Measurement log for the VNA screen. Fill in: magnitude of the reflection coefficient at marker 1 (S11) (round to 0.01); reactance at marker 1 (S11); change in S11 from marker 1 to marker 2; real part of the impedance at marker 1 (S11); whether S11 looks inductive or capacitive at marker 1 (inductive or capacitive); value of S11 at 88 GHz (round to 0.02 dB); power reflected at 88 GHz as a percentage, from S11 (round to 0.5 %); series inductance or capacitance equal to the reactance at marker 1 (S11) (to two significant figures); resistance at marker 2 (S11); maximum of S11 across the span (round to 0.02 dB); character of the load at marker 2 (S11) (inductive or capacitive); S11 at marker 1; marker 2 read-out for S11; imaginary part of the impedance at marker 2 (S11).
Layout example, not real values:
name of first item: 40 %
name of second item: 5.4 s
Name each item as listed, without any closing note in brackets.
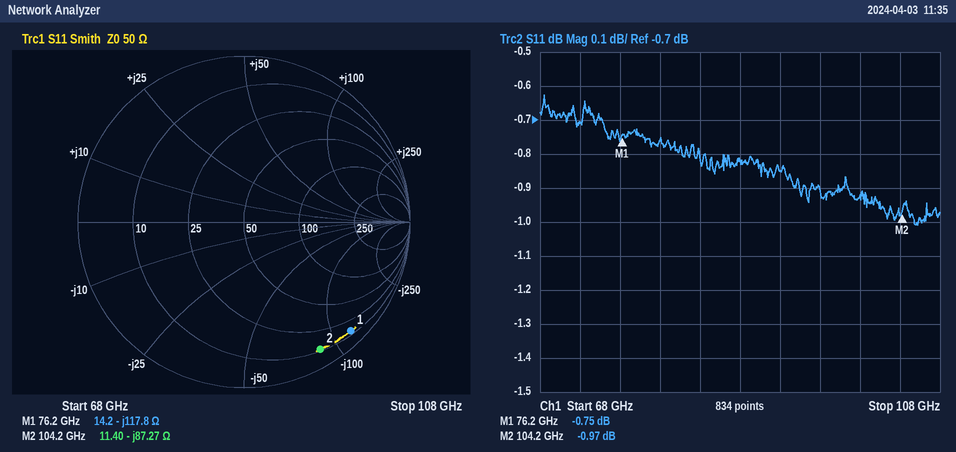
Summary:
magnitude of the reflection coefficient at marker 1 (S11): 0.92
reactance at marker 1: -117.8 Ω
change in S11 from marker 1 to marker 2: -0.22 dB
real part of the impedance at marker 1: 14.2 Ω
whether S11 looks inductive or capacitive at marker 1: capacitive
value of S11 at 88 GHz: -0.82 dB
power reflected at 88 GHz as a percentage, from S11: 83.0 %
series inductance or capacitance equal to the reactance at marker 1 (S11): 18 fF
resistance at marker 2: 11.40 Ω
maximum of S11 across the span: -0.62 dB
character of the load at marker 2 (S11): capacitive
S11 at marker 1: -0.75 dB
marker 2 read-out for S11: -0.97 dB
imaginary part of the impedance at marker 2: -87.27 Ω
